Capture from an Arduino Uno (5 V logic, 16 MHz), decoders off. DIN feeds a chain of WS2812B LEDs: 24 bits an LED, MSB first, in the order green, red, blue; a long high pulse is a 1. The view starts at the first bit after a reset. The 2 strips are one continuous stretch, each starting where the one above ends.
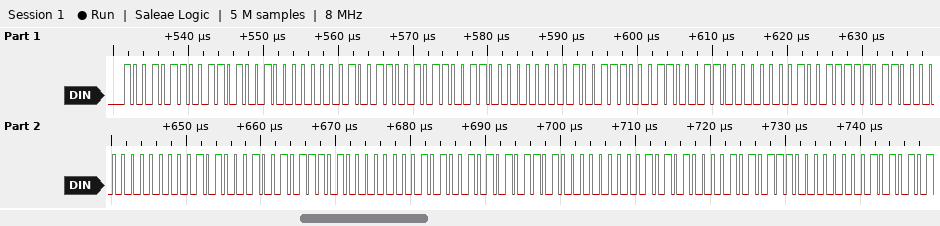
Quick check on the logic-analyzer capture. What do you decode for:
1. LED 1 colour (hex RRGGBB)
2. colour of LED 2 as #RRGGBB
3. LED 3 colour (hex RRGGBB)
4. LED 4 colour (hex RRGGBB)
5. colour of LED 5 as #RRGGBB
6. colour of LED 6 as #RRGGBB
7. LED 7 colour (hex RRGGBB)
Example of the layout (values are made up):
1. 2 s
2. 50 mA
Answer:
1. #699600
2. #669900
3. #639C00
4. #609F00
5. #5DA200
6. #5AA500
7. #57A800
